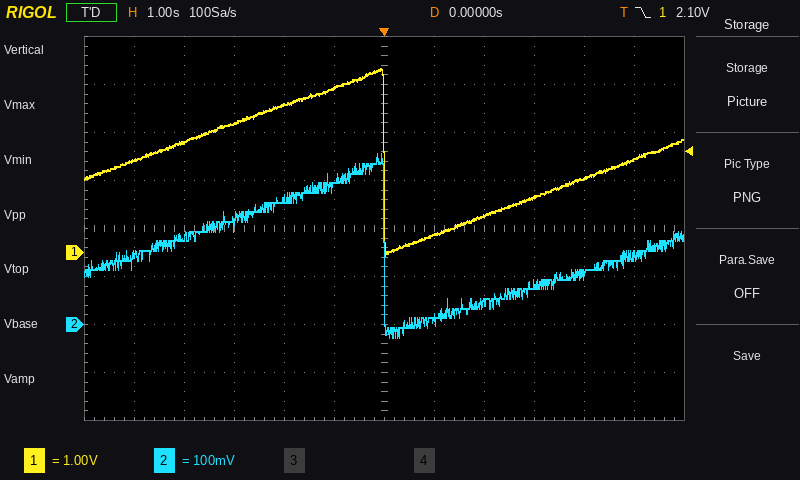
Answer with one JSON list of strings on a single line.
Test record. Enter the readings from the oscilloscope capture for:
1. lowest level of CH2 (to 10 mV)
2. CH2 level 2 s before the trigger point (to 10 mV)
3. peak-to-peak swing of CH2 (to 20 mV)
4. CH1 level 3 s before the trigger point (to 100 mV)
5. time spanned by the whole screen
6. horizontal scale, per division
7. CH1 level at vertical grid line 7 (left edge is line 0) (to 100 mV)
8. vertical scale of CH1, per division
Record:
["-30 mV", "260 mV", "380 mV", "2.7 V", "12 s", "1 s", "400 mV", "1 V"]
